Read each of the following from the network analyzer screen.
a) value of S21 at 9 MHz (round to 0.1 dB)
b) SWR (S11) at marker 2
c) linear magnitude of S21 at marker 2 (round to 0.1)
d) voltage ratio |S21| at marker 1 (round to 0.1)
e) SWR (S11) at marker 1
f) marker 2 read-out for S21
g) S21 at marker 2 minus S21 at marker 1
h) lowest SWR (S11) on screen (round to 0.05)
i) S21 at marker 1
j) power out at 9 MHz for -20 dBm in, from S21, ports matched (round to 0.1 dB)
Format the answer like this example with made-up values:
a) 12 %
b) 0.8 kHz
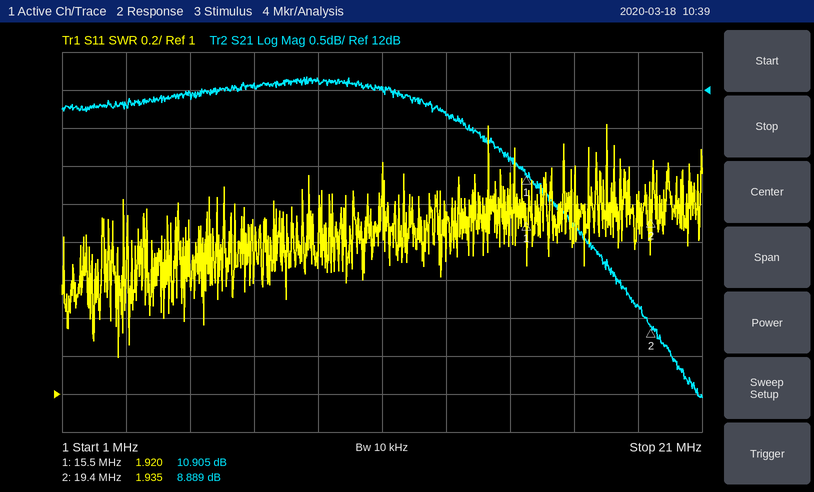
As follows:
a) 12.1 dB
b) 1.935
c) 2.8
d) 3.5
e) 1.920
f) 8.889 dB
g) -2.016 dB
h) 1.20
i) 10.905 dB
j) -7.9 dBm
